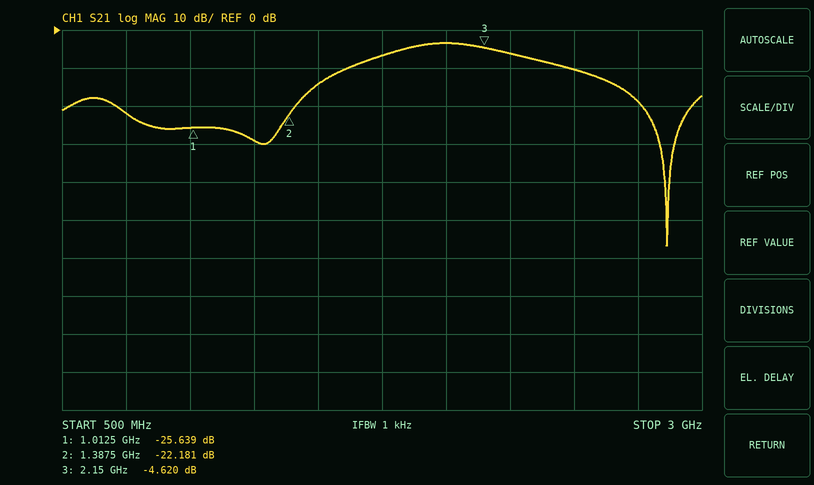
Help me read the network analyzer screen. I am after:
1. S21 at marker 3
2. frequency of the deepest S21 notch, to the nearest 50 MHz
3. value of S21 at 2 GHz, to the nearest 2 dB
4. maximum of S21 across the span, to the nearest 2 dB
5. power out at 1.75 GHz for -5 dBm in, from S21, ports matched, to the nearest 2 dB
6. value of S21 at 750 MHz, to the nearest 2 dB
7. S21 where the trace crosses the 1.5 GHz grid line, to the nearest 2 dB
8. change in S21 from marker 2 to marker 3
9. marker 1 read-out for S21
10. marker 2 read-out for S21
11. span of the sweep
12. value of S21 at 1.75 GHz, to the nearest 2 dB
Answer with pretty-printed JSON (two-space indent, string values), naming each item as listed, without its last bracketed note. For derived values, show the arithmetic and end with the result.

{
  "S21 at marker 3": "-4.620 dB",
  "frequency of the deepest S21 notch, to the nearest 50 MHz": "2.85 GHz",
  "value of S21 at 2 GHz, to the nearest 2 dB": "-4 dB",
  "maximum of S21 across the span, to the nearest 2 dB": "-4 dB",
  "power out at 1.75 GHz for -5 dBm in, from S21, ports matched, to the nearest 2 dB": "-5 dBm + (-6 dB) = -12 dBm",
  "value of S21 at 750 MHz, to the nearest 2 dB": "-22 dB",
  "S21 where the trace crosses the 1.5 GHz grid line, to the nearest 2 dB": "-14 dB",
  "change in S21 from marker 2 to marker 3": "-4.62 − (-22.181) = 17.561 dB",
  "marker 1 read-out for S21": "-25.639 dB",
  "marker 2 read-out for S21": "-22.181 dB",
  "span of the sweep": "2.5 GHz",
  "value of S21 at 1.75 GHz, to the nearest 2 dB": "-6 dB"
}
